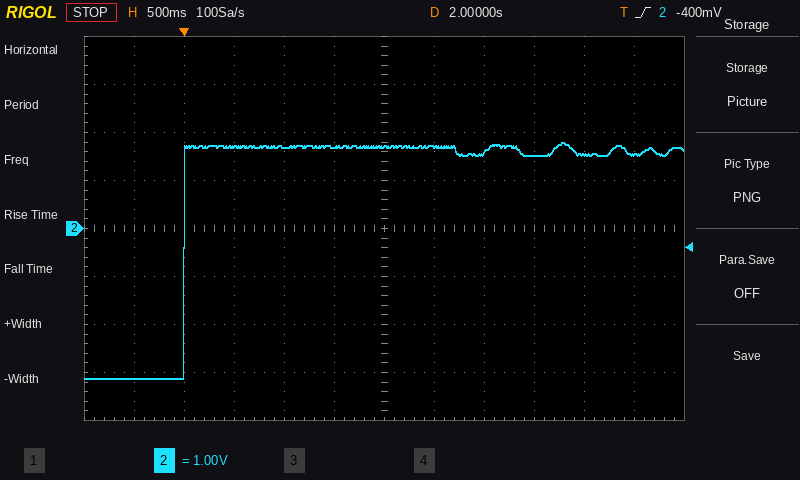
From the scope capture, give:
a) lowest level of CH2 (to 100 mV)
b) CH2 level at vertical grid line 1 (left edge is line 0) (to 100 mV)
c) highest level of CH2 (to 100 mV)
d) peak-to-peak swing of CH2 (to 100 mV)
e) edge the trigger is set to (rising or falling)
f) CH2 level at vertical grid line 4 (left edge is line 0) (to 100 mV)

-3.1 V
-3.1 V
1.8 V
4.9 V
rising
1.7 V
